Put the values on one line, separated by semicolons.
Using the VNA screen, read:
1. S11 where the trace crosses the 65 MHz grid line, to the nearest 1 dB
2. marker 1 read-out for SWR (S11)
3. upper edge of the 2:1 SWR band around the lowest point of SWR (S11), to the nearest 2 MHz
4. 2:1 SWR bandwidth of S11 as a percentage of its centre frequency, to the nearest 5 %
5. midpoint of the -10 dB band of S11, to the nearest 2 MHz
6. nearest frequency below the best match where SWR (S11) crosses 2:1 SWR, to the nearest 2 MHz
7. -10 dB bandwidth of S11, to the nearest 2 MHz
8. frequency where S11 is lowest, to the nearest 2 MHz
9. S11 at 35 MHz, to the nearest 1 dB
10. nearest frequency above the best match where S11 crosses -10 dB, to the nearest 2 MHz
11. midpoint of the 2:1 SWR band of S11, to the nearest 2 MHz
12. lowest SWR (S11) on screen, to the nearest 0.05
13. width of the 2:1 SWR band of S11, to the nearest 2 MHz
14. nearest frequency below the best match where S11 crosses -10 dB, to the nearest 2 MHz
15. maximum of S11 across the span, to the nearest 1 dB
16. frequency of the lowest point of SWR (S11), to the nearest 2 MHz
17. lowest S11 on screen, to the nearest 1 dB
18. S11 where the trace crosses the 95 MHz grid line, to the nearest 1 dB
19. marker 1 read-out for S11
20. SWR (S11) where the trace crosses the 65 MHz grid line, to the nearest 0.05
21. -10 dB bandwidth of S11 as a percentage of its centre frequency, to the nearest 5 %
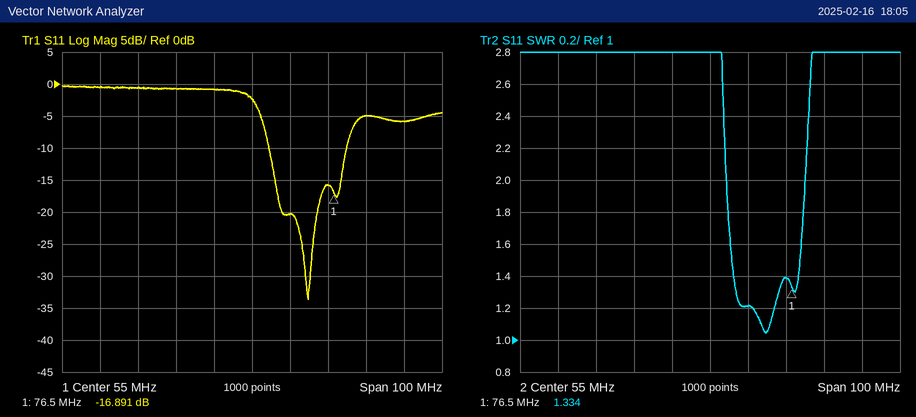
-20 dB; 1.334; 80 MHz; 30 %; 70 MHz; 60 MHz; 20 MHz; 70 MHz; -1 dB; 80 MHz; 70 MHz; 1.05; 20 MHz; 60 MHz; 0 dB; 70 MHz; -34 dB; -6 dB; -16.891 dB; 1.20; 30 %
